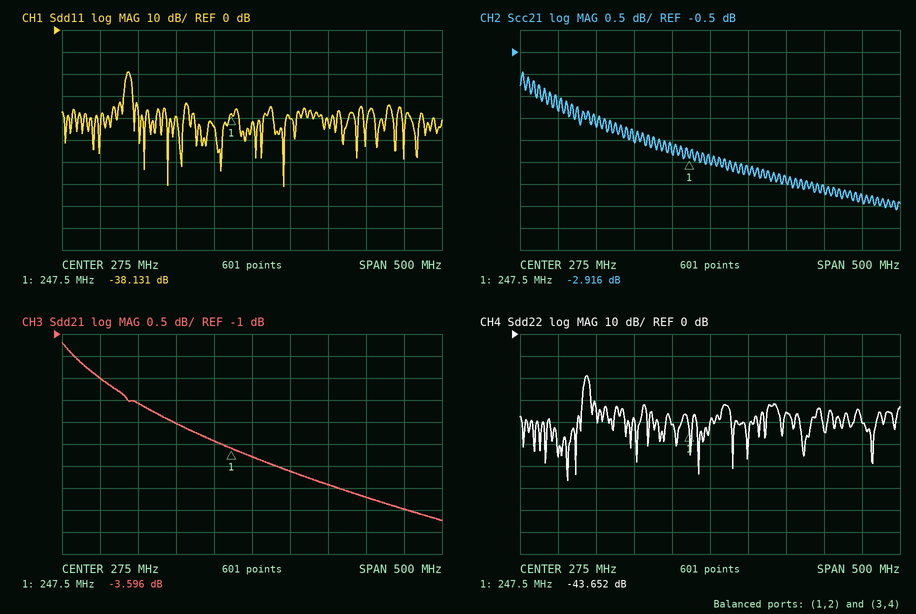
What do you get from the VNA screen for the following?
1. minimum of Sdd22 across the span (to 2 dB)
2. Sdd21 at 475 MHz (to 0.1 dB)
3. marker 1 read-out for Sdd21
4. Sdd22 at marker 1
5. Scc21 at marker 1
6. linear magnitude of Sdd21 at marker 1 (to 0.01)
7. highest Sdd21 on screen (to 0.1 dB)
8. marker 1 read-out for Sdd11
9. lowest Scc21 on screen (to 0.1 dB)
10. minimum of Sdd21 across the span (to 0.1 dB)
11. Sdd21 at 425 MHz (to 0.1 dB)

-66 dB
-5.0 dB
-3.596 dB
-43.652 dB
-2.916 dB
0.66
-1.2 dB
-38.131 dB
-4.1 dB
-5.2 dB
-4.7 dB
